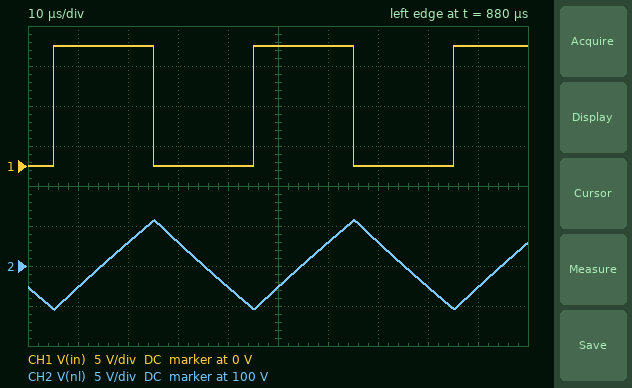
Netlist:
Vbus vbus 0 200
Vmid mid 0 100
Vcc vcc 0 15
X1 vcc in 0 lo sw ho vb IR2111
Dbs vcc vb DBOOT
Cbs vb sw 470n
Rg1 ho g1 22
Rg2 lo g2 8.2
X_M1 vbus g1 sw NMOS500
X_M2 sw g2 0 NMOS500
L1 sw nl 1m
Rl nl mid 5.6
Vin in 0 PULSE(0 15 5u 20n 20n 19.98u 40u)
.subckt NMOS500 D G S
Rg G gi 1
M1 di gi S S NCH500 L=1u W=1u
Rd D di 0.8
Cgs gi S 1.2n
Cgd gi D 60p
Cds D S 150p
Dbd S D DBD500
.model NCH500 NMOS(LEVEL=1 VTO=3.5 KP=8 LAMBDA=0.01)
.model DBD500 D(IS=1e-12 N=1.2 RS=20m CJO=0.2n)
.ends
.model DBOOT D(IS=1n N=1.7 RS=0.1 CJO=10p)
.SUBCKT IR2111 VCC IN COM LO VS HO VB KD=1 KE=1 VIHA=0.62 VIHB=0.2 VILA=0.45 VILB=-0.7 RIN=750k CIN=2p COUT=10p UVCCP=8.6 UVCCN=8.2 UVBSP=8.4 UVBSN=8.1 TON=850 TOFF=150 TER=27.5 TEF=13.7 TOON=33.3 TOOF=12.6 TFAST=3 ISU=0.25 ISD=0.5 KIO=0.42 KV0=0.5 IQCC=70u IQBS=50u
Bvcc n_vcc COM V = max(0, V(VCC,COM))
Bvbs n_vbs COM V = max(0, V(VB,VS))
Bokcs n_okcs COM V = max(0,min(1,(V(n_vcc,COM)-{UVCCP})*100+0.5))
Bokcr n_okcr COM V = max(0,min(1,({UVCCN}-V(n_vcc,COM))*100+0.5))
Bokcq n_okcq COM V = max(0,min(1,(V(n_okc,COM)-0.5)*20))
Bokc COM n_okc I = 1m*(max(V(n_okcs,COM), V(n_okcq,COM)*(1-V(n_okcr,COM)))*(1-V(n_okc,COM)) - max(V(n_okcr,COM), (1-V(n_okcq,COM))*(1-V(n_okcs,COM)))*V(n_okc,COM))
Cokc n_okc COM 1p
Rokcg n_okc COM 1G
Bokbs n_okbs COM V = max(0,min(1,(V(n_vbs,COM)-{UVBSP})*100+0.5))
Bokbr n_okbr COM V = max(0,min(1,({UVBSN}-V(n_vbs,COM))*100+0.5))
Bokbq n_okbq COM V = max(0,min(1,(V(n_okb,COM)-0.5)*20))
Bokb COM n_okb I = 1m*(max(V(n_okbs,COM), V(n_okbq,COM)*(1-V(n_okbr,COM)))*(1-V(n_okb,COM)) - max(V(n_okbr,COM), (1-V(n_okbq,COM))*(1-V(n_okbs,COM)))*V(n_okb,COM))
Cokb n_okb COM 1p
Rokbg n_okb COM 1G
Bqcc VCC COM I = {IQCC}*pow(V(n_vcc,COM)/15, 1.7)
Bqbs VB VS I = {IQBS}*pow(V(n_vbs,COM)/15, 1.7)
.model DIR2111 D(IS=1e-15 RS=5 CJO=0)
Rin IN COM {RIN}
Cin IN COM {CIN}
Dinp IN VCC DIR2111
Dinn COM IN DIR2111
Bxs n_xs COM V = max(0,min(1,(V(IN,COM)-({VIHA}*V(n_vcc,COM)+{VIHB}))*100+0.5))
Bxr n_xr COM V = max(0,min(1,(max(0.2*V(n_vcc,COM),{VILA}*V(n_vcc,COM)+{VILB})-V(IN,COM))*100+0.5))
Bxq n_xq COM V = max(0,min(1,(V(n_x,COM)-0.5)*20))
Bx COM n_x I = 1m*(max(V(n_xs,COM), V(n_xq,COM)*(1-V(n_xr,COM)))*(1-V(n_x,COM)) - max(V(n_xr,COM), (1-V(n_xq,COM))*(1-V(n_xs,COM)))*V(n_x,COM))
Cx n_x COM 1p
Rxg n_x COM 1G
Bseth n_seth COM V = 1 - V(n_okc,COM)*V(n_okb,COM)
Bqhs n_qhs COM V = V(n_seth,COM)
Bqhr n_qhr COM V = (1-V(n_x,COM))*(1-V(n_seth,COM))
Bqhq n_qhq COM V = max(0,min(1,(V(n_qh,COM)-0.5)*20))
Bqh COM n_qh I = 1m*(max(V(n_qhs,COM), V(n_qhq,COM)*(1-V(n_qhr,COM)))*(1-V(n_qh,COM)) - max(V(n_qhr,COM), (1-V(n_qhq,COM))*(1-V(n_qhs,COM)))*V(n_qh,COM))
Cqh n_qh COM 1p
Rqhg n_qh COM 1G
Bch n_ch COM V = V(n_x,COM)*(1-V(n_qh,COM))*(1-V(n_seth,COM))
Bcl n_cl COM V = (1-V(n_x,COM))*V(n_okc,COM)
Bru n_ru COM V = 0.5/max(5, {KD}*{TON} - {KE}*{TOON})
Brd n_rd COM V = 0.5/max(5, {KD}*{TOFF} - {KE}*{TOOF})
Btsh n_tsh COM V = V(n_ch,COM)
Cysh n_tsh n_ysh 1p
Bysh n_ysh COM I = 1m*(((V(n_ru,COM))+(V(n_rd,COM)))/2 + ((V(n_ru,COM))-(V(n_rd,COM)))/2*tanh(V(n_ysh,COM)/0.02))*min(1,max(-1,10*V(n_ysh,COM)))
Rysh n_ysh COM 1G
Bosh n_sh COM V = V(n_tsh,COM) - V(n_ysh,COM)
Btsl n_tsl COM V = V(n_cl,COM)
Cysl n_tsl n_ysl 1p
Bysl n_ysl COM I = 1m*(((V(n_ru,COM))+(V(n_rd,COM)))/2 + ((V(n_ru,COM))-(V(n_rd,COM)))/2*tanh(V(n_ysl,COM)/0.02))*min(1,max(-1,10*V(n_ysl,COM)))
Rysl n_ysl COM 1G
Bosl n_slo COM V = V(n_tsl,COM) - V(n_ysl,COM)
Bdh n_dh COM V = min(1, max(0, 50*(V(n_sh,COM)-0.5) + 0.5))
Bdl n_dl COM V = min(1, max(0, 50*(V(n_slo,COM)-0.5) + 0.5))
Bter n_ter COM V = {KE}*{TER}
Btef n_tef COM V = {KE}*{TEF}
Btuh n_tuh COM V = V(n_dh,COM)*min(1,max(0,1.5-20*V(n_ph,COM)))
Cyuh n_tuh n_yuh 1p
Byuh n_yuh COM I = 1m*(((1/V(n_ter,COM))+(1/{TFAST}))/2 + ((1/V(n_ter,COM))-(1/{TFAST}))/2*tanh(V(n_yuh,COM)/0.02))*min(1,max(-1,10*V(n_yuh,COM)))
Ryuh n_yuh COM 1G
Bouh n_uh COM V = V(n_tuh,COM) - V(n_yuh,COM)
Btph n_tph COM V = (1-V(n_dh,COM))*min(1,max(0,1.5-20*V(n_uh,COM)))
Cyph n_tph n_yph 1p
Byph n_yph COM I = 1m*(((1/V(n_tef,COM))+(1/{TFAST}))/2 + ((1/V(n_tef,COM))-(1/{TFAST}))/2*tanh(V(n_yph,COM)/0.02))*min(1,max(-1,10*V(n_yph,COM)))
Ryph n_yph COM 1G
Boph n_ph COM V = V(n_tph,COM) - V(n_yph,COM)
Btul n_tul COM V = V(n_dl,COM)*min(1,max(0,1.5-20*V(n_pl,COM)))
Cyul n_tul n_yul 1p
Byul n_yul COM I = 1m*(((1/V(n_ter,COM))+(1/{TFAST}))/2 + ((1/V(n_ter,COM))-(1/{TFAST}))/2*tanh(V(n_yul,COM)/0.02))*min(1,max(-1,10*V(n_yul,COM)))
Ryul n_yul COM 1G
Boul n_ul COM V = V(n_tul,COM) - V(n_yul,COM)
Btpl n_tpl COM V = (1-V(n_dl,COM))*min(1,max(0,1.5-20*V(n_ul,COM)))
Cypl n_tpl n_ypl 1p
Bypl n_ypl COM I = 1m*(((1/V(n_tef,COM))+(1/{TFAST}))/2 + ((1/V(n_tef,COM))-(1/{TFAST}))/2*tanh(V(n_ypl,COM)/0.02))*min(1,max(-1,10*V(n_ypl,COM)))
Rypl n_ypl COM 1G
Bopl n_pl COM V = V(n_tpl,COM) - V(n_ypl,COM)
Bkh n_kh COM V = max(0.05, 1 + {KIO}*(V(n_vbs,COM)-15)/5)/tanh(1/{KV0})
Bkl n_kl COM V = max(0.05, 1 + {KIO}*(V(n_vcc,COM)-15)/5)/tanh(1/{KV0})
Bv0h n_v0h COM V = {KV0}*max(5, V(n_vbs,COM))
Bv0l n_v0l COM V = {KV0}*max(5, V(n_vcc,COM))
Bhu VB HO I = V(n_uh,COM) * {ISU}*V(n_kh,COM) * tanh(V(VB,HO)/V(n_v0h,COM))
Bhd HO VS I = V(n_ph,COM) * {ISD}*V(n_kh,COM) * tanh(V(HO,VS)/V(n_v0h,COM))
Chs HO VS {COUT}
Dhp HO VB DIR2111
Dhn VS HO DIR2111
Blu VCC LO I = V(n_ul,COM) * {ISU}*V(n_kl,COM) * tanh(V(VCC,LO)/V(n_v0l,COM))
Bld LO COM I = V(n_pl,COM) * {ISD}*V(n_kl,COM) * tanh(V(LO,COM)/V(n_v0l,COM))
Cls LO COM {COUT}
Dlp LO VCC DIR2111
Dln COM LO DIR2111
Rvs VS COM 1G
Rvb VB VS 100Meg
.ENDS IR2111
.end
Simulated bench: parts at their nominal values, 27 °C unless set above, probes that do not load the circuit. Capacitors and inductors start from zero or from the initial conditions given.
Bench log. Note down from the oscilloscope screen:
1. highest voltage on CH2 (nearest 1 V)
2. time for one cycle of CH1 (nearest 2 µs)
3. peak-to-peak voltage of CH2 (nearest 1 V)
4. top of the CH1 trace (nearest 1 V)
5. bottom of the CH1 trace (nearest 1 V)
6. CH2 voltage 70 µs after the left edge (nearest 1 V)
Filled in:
106 V
40 µs
11 V
15 V
0 V
103 V
